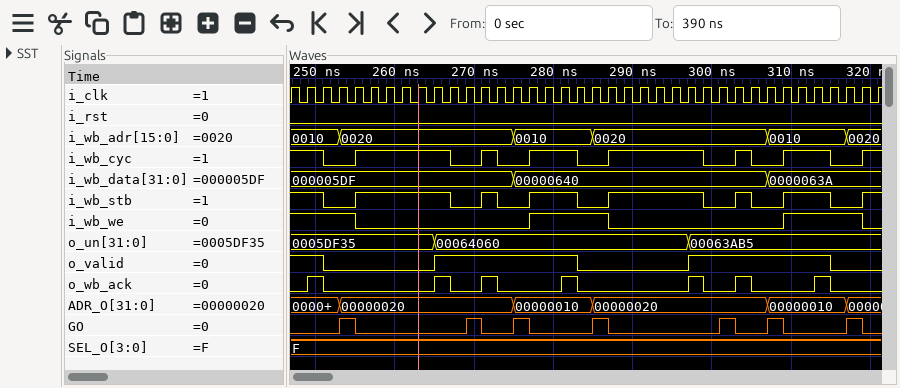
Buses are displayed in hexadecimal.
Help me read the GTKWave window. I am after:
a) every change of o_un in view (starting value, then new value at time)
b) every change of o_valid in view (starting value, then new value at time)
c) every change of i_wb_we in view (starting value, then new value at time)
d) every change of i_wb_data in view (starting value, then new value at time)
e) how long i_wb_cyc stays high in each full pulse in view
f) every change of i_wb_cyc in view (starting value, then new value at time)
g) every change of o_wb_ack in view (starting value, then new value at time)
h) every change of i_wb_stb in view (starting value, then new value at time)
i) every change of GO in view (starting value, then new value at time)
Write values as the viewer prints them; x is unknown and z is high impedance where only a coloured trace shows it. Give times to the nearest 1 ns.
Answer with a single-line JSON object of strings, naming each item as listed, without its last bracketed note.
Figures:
{"every change of o_un in view": "0005DF35, 00064060 at 265 ns, 00063AB5 at 297 ns", "every change of o_valid in view": "1, 0 at 251 ns, 1 at 265 ns, 0 at 283 ns, 1 at 297 ns, 0 at 315 ns", "every change of i_wb_we in view": "1, 0 at 255 ns, 1 at 277 ns, 0 at 287 ns, 1 at 309 ns, 0 at 319 ns", "every change of i_wb_data in view": "000005DF, 00000640 at 275 ns, 0000063A at 307 ns", "how long i_wb_cyc stays high in each full pulse in view": "12 ns, 2 ns, 6 ns, 12 ns, 2 ns, 6 ns", "every change of i_wb_cyc in view": "1, 0 at 251 ns, 1 at 255 ns, 0 at 267 ns, 1 at 271 ns, 0 at 273 ns, 1 at 277 ns, 0 at 283 ns, 1 at 287 ns, 0 at 299 ns, 1 at 303 ns, 0 at 305 ns, 1 at 309 ns, 0 at 315 ns, 1 at 319 ns", "every change of o_wb_ack in view": "0, 1 at 249 ns, 0 at 251 ns, 1 at 265 ns, 0 at 267 ns, 1 at 271 ns, 0 at 273 ns, 1 at 281 ns, 0 at 283 ns, 1 at 297 ns, 0 at 299 ns, 1 at 303 ns, 0 at 305 ns, 1 at 313 ns, 0 at 315 ns", "every change of i_wb_stb in view": "1, 0 at 251 ns, 1 at 255 ns, 0 at 267 ns, 1 at 271 ns, 0 at 273 ns, 1 at 277 ns, 0 at 283 ns, 1 at 287 ns, 0 at 299 ns, 1 at 303 ns, 0 at 305 ns, 1 at 309 ns, 0 at 315 ns, 1 at 319 ns", "every change of GO in view": "0, 1 at 253 ns, 0 at 255 ns, 1 at 269 ns, 0 at 271 ns, 1 at 275 ns, 0 at 277 ns, 1 at 285 ns, 0 at 287 ns, 1 at 301 ns, 0 at 303 ns, 1 at 307 ns, 0 at 309 ns, 1 at 317 ns, 0 at 319 ns"}
